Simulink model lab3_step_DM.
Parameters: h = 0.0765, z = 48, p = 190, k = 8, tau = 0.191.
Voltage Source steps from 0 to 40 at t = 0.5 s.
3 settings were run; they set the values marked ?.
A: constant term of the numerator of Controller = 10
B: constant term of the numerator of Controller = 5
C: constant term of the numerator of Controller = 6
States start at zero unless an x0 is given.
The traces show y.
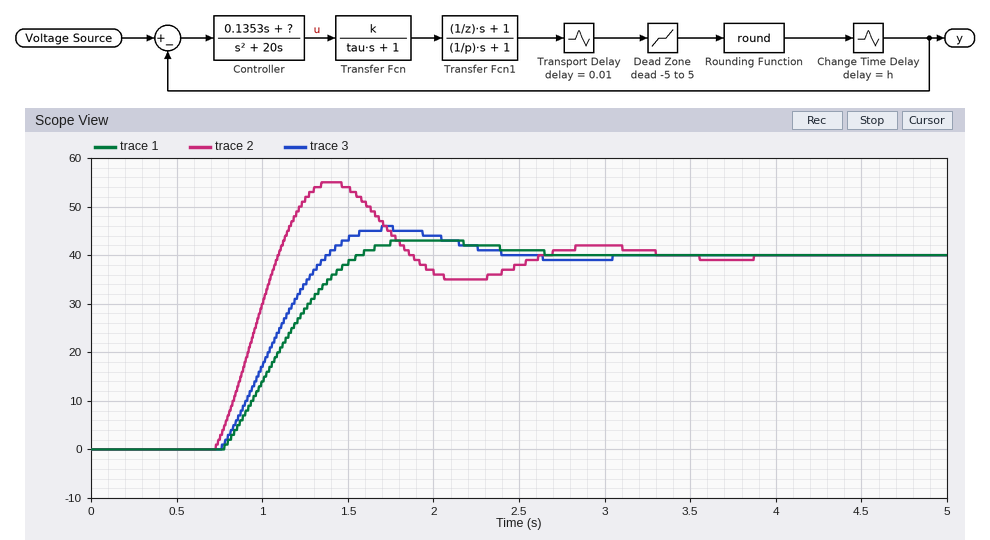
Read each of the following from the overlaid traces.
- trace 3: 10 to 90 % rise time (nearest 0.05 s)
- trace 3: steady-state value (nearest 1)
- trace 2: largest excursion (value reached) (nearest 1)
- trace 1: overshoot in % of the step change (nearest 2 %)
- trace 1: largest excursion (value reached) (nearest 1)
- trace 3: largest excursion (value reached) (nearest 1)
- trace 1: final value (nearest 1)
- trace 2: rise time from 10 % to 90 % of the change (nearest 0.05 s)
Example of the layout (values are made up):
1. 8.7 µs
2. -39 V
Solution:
1. 0.45 s
2. 40
3. 55
4. 8 %
5. 43
6. 46
7. 40
8. 0.30 s
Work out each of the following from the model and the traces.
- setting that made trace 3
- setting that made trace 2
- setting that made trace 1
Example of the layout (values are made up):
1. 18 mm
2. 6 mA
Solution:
1. C
2. A
3. B
